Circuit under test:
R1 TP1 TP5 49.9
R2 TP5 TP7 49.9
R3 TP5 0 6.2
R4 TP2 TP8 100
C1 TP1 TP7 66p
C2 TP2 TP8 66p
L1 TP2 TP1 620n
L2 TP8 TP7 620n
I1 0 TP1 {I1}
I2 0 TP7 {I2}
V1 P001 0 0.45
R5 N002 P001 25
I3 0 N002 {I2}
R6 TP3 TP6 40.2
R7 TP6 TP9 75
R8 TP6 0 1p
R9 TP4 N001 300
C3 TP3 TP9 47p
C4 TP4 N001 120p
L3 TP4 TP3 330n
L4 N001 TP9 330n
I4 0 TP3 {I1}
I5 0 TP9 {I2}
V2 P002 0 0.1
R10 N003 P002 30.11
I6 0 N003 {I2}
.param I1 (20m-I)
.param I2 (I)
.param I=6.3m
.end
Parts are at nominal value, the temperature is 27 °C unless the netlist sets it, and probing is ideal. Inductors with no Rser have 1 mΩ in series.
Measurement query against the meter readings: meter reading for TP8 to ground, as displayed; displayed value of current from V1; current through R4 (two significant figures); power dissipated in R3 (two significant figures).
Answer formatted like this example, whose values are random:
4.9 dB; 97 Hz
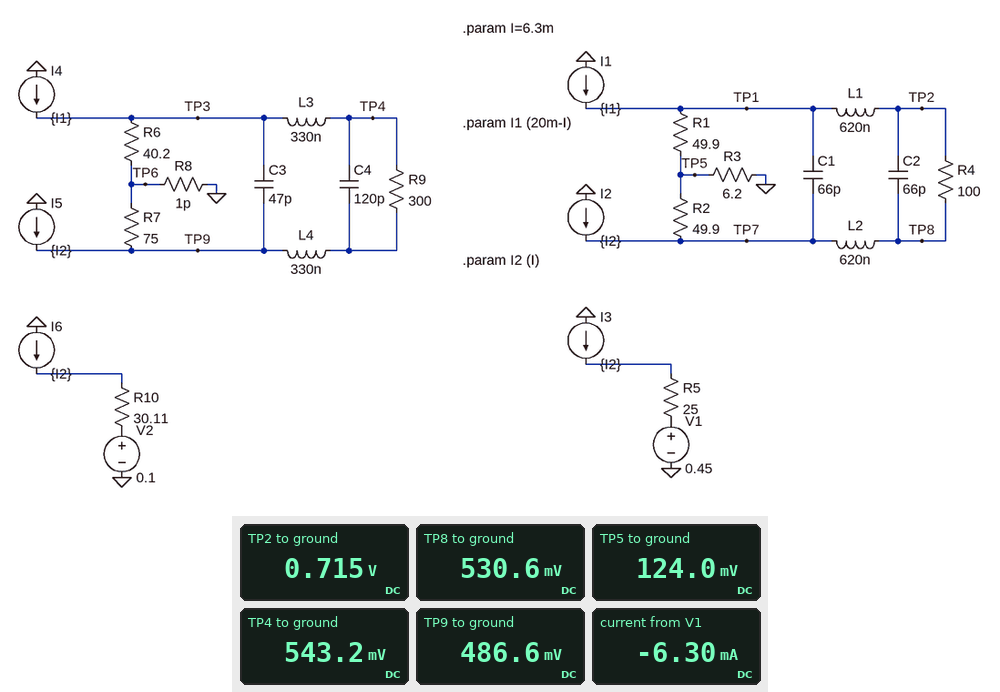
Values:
530.6 mV; -6.30 mA; 1.8 mA; 2.5 mW
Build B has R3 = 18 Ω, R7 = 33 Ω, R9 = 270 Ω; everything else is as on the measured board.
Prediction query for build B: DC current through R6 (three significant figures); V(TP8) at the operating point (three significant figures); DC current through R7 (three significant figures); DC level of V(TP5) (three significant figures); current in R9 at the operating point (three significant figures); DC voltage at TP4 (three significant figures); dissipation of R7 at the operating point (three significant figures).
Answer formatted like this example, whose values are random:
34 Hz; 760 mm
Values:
12.7 mA; 767 mV; 7.30 mA; 360 mV; 999 µA; 511 mV; 1.76 mW
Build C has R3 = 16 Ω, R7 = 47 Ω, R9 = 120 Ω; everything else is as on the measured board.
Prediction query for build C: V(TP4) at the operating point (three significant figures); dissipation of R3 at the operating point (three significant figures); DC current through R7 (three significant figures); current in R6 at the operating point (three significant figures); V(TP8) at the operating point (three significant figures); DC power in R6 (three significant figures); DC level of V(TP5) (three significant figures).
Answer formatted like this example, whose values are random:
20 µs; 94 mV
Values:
501 mV; 6.40 mW; 7.53 mA; 12.5 mA; 727 mV; 6.25 mW; 320 mV
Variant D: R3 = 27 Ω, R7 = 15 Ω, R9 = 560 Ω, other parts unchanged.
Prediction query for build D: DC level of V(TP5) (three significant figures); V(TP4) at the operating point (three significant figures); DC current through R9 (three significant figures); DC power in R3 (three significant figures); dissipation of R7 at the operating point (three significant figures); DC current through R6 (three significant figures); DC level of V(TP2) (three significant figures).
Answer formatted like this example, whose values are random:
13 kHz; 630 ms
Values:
540 mV; 521 mV; 742 µA; 10.8 mW; 744 µW; 13.0 mA; 1.13 V
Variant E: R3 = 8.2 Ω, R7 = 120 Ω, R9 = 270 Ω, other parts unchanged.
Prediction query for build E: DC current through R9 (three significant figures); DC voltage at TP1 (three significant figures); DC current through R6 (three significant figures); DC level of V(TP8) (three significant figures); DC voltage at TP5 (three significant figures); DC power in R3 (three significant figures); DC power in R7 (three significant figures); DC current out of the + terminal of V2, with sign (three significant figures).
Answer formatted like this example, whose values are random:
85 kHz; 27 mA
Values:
477 µA; 755 mV; 14.2 mA; 571 mV; 164 mV; 3.28 mW; 4.07 mW; -6.30 mA
